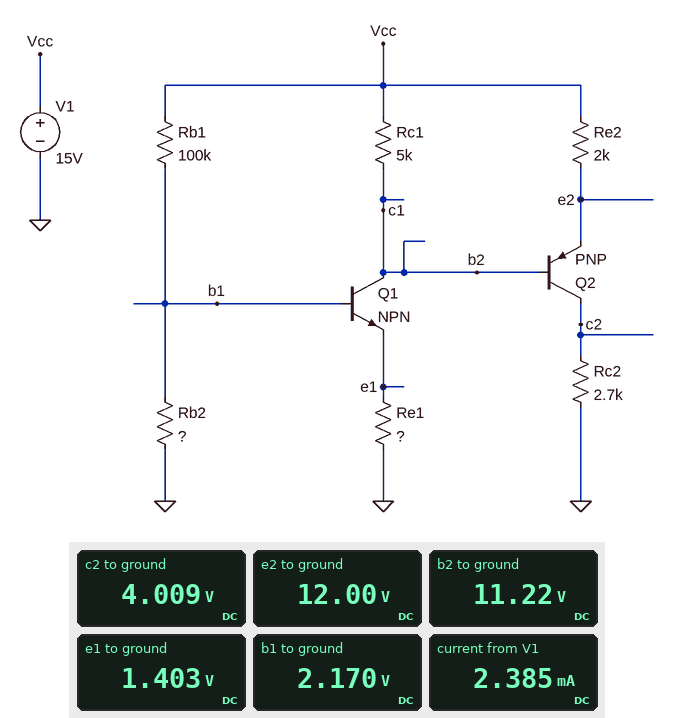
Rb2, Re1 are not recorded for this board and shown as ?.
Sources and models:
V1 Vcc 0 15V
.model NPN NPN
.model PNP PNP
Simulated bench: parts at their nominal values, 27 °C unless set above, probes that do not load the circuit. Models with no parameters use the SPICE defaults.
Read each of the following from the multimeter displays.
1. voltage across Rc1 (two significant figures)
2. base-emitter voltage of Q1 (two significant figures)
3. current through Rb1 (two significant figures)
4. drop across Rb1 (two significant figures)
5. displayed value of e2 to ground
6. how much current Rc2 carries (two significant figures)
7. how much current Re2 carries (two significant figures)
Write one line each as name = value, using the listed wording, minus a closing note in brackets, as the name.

voltage across Rc1 = 3.8 V
base-emitter voltage of Q1 = 770 mV
current through Rb1 = 130 µA
drop across Rb1 = 13 V
displayed value of e2 to ground = 12.00 V
how much current Rc2 carries = 1.5 mA
how much current Re2 carries = 1.5 mA
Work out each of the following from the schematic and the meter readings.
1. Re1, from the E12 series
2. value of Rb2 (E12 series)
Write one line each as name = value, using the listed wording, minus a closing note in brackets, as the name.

Re1, from the E12 series = 1.8 kΩ
value of Rb2 = 18 kΩ
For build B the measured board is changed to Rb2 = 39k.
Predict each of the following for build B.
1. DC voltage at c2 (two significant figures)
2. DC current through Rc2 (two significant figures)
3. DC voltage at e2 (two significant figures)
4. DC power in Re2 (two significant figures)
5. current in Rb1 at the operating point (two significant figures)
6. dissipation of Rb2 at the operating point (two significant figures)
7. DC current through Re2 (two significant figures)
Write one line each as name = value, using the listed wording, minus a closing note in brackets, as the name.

DC voltage at c2 = 8.4 V
DC current through Rc2 = 3.1 mA
DC voltage at e2 = 8.5 V
DC power in Re2 = 21 mW
current in Rb1 at the operating point = 110 µA
dissipation of Rb2 at the operating point = 360 µW
DC current through Re2 = 3.3 mA
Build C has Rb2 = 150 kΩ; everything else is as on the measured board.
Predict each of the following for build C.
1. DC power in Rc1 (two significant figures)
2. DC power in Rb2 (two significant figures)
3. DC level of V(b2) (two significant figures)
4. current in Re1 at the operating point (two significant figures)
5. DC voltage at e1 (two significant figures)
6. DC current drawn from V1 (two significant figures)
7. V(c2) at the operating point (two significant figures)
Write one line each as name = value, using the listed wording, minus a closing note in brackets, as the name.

DC power in Rc1 = 16 mW
DC power in Rb2 = 300 µW
DC level of V(b2) = 6.1 V
current in Re1 at the operating point = 3.3 mA
DC voltage at e1 = 5.9 V
DC current drawn from V1 = 5.9 mA
V(c2) at the operating point = 6.9 V
